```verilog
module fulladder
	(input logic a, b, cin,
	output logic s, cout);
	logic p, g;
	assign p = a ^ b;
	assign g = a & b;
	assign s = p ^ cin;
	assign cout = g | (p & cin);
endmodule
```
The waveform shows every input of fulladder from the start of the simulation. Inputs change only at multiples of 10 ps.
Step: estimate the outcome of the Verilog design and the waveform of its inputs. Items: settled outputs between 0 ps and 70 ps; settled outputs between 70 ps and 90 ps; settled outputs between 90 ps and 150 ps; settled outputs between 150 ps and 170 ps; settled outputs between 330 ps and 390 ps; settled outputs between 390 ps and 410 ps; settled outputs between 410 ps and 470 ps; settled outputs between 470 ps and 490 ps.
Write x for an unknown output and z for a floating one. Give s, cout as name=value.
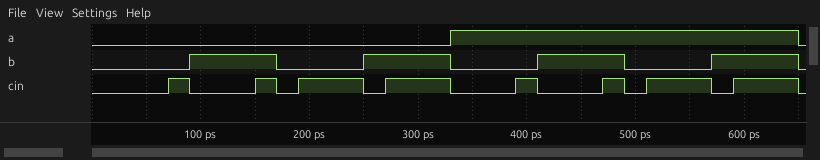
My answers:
s=0, cout=0
s=1, cout=0
s=1, cout=0
s=0, cout=1
s=1, cout=0
s=0, cout=1
s=0, cout=1
s=1, cout=1
